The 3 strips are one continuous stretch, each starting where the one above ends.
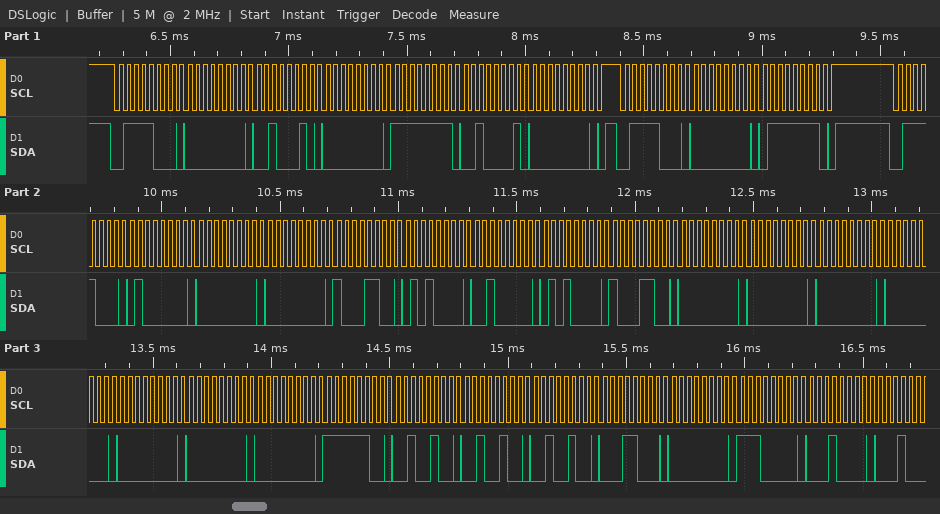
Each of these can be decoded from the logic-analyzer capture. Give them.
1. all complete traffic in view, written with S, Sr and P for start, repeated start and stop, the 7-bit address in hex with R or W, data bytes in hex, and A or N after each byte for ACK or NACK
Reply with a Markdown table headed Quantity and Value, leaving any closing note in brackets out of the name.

| Quantity | Value |
|---|---|
| all complete traffic in view, written with S, Sr and P for start, repeated start and stop, the 7-bit address in hex with R or W, data bytes in hex, and A or N after each byte for ACK or NACK | S 3CW A 00 A 22 A 00 A FF A 21 A 00 A P S 3CW A 00 A 7F A P S 3CW A 40 A 00 A 00 A 8C A 50 A 20 A 50 A 8C A 00 A 00 A 00 A 00 A 00 A 00 A 00 A FC A 24 A 24 A 24 A 18 A 00 A E0 A 10 A |
